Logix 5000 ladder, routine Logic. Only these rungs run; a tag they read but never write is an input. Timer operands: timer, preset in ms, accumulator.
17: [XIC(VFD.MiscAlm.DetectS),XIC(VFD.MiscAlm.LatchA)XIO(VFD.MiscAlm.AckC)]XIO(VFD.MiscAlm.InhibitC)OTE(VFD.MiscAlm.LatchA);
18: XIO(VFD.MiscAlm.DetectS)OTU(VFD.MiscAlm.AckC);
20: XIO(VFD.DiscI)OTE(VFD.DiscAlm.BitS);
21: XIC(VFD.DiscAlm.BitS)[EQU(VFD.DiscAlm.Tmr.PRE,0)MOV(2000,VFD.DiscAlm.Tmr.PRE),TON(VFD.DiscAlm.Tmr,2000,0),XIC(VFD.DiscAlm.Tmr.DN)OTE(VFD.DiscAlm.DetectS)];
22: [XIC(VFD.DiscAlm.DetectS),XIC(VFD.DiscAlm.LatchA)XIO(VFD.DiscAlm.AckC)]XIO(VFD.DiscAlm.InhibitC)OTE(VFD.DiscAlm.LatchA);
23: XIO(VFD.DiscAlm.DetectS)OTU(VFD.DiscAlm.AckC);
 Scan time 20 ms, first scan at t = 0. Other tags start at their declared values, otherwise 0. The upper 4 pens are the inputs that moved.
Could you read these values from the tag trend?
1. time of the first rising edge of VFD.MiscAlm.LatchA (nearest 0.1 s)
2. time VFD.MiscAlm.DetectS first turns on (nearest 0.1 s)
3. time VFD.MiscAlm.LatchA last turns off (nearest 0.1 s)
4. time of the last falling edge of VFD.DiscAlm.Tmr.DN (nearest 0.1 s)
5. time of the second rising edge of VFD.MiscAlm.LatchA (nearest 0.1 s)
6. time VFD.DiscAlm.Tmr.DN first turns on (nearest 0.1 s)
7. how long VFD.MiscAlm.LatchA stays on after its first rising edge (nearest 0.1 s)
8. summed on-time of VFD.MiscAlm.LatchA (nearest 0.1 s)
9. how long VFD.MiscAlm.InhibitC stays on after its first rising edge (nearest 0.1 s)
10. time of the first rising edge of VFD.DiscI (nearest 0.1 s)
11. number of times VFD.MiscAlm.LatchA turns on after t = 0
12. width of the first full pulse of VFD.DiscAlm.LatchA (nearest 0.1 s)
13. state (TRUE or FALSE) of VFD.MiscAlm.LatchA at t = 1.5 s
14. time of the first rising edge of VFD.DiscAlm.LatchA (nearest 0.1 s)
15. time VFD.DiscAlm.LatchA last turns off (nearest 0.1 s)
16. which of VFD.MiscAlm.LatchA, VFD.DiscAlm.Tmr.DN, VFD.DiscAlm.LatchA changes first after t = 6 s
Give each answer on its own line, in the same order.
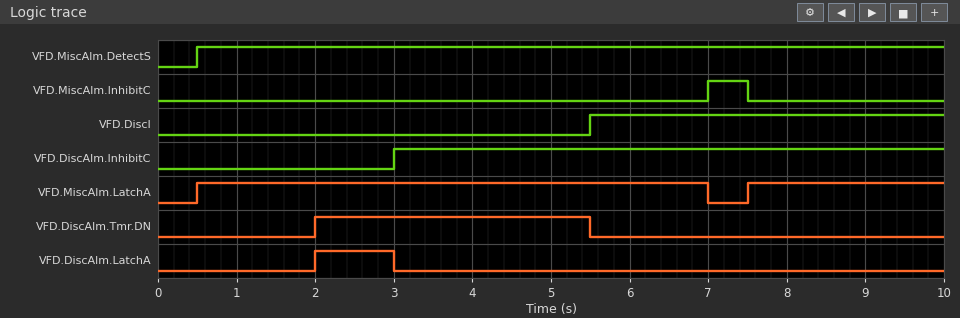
0.5 s
0.5 s
7.0 s
5.5 s
7.5 s
2.0 s
6.5 s
9.0 s
0.5 s
5.5 s
2
1.0 s
TRUE
2.0 s
3.0 s
VFD.MiscAlm.LatchA
